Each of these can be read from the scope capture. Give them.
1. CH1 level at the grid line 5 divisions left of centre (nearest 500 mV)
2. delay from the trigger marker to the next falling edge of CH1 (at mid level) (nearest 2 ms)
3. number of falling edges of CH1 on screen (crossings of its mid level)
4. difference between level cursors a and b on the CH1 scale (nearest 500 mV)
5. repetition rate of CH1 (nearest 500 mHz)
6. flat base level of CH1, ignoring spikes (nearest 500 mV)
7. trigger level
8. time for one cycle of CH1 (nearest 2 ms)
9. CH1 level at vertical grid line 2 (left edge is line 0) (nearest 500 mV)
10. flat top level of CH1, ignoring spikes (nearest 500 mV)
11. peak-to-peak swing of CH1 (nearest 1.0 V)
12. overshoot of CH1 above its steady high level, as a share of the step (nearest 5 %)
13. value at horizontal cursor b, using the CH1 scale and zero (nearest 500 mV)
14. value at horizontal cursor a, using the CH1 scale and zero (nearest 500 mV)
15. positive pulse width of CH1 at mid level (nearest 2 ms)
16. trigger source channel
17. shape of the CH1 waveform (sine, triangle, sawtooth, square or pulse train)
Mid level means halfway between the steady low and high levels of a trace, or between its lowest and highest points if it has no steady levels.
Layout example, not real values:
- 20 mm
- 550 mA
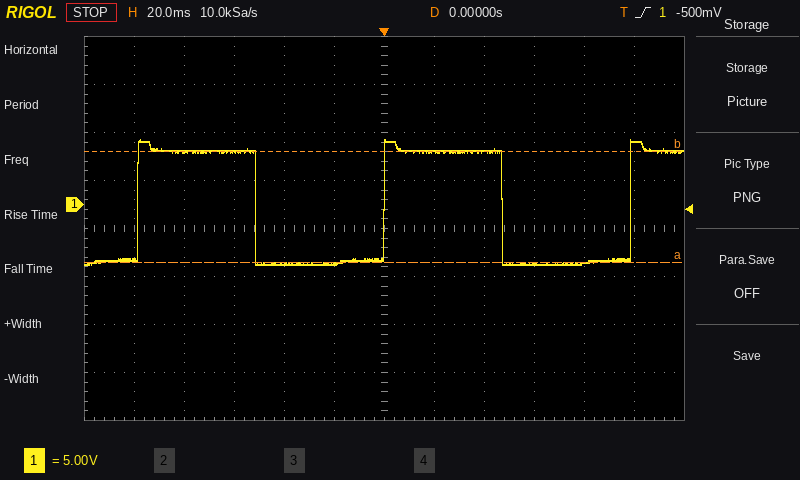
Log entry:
- -5.5 V
- 48 ms
- 2
- 11.5 V
- 10.0 Hz
- -6.0 V
- -500 mV
- 98 ms
- 5.5 V
- 5.5 V
- 13.0 V
- 10 %
- 5.5 V
- -6.0 V
- 48 ms
- CH1
- square
